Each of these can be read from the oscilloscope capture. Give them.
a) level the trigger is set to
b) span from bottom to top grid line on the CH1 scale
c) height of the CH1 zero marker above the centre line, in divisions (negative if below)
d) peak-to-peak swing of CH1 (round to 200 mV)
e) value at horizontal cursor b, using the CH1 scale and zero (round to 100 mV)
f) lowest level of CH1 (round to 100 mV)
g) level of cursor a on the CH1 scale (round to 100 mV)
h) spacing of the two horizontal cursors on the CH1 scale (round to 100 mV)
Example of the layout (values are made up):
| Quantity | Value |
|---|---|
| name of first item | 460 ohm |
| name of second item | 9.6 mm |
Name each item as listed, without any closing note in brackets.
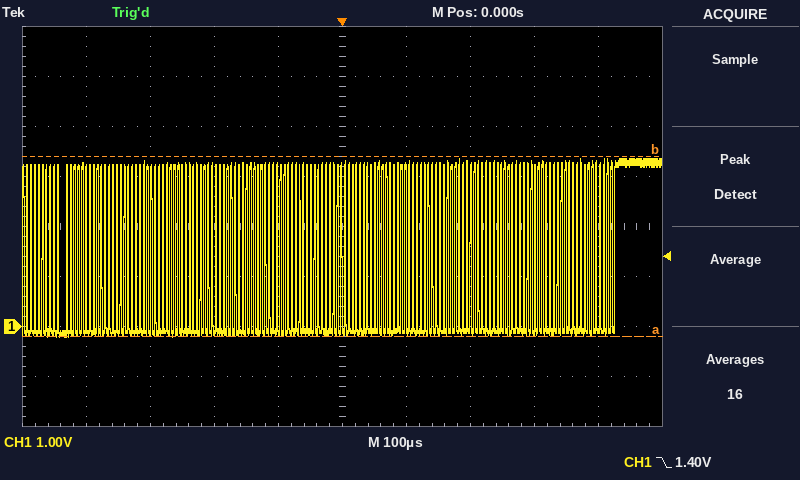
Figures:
| Quantity | Value |
|---|---|
| level the trigger is set to | 1.40 V |
| span from bottom to top grid line on the CH1 scale | 8 V |
| height of the CH1 zero marker above the centre line, in divisions | -2.0 div |
| peak-to-peak swing of CH1 | 3.6 V |
| value at horizontal cursor b, using the CH1 scale and zero | 3.4 V |
| lowest level of CH1 | -200 mV |
| level of cursor a on the CH1 scale | -200 mV |
| spacing of the two horizontal cursors on the CH1 scale | 3.6 V |
